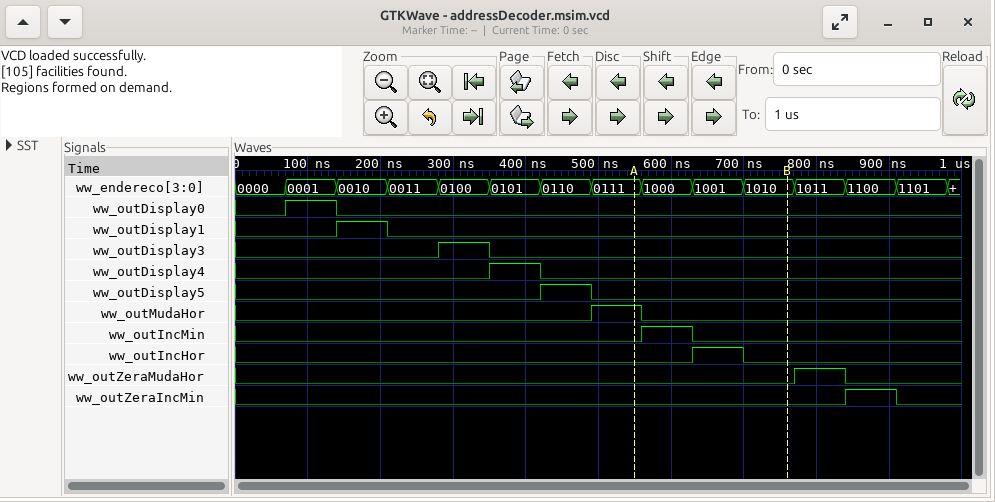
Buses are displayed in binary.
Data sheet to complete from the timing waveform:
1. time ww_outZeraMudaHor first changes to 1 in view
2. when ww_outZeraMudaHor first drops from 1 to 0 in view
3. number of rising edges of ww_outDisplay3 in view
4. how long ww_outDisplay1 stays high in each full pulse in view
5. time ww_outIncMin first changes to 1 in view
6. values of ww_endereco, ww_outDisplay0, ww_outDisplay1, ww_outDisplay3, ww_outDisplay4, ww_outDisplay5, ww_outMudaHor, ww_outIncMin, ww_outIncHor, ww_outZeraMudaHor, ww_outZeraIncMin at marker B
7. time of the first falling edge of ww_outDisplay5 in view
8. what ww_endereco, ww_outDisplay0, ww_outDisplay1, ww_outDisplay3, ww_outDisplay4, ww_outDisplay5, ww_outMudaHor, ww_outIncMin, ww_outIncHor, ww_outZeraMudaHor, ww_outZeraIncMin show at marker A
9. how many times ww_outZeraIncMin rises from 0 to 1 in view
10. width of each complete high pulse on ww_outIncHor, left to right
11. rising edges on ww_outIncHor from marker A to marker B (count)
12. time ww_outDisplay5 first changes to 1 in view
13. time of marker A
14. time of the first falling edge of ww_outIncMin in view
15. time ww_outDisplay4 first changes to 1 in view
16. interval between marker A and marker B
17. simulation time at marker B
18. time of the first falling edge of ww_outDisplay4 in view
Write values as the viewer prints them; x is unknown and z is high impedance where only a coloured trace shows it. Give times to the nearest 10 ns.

770 ns
840 ns
1
70 ns
560 ns
ww_endereco=1010, ww_outDisplay0=0, ww_outDisplay1=0, ww_outDisplay3=0, ww_outDisplay4=0, ww_outDisplay5=0, ww_outMudaHor=0, ww_outIncMin=0, ww_outIncHor=0, ww_outZeraMudaHor=0, ww_outZeraIncMin=0
490 ns
ww_endereco=0111, ww_outDisplay0=0, ww_outDisplay1=0, ww_outDisplay3=0, ww_outDisplay4=0, ww_outDisplay5=0, ww_outMudaHor=1, ww_outIncMin=0, ww_outIncHor=0, ww_outZeraMudaHor=0, ww_outZeraIncMin=0
1
70 ns
1
420 ns
550 ns
630 ns
350 ns
210 ns
760 ns
420 ns
